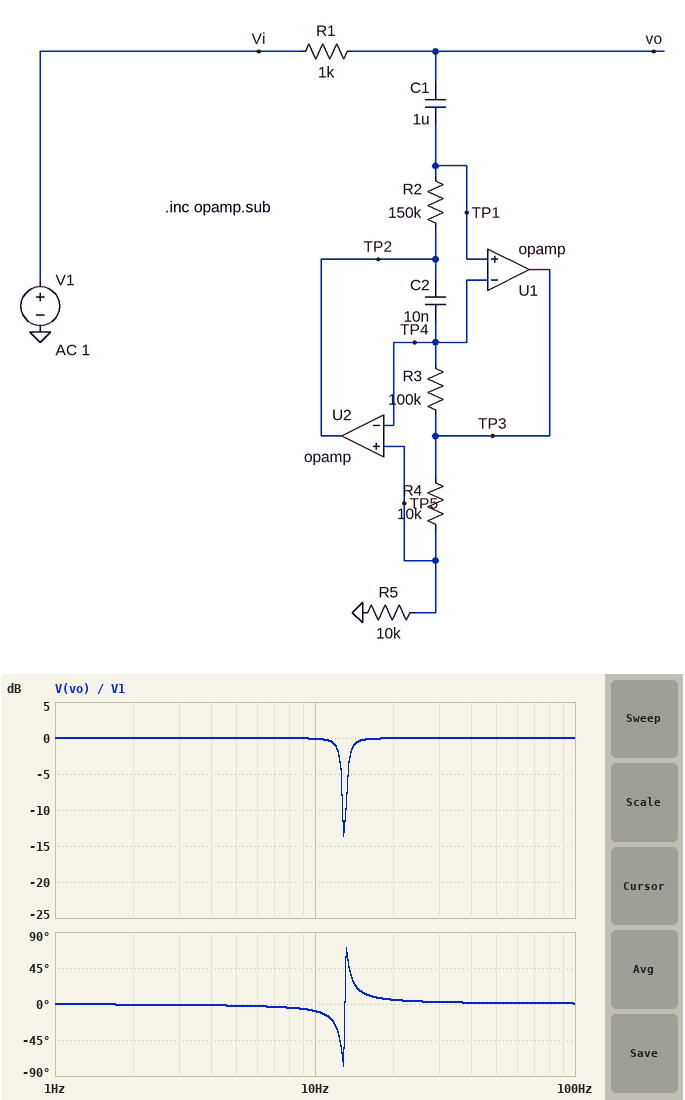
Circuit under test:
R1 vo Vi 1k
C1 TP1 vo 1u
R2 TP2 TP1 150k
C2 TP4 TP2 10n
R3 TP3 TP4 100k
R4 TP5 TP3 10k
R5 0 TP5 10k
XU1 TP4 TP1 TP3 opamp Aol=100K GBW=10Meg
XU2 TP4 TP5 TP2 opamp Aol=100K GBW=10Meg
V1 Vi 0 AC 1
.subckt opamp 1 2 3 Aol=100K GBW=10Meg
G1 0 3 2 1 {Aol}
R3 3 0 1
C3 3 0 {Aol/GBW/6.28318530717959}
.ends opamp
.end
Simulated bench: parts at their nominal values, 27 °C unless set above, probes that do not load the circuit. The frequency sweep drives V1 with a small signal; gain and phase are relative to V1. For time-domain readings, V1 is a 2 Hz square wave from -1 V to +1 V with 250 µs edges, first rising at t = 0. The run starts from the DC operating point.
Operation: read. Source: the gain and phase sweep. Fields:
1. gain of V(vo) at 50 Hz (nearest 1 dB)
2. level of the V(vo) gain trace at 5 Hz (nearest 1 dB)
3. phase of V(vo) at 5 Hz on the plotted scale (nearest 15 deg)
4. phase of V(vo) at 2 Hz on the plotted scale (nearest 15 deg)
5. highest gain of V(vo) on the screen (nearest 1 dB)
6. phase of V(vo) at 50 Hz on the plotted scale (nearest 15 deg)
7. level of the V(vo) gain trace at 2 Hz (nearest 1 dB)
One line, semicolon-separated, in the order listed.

0 dB; 0 dB; 0 deg; 0 deg; 0 dB; 0 deg; 0 dB
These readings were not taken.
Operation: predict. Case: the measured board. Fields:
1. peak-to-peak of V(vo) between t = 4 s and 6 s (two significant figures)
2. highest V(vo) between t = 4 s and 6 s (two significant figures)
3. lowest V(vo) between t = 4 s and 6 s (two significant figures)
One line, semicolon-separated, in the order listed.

2.2 V; 1.1 V; -1.1 V
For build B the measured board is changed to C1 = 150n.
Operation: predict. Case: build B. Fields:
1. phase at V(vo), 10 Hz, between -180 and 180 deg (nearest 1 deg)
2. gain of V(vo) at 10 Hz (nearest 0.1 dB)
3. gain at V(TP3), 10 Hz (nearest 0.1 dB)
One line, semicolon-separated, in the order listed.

-1 deg; 0 dB; -14.2 dB
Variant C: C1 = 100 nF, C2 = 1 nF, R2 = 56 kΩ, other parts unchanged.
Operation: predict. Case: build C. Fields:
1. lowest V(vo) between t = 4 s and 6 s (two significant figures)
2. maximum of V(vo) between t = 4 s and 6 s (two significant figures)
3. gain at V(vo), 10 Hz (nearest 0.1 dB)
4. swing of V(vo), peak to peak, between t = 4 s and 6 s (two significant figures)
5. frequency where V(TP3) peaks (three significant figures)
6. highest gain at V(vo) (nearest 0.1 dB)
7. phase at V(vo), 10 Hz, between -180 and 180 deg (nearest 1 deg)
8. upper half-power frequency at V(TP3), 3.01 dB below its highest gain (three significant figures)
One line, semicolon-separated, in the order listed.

-1.2 V; 1.2 V; 0 dB; 2.4 V; 214 Hz; 0 dB; 0 deg; 230 Hz
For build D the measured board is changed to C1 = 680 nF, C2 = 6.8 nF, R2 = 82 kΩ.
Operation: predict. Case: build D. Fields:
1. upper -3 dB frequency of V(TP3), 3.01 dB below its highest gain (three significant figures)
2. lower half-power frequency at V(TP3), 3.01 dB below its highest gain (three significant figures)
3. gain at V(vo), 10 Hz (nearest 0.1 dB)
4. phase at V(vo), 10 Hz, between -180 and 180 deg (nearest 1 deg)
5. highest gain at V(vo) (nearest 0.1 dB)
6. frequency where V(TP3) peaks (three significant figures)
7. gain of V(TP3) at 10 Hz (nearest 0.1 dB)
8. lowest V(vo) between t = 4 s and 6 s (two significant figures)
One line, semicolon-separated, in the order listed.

27.5 Hz; 24.6 Hz; 0 dB; -3 deg; 0 dB; 25.9 Hz; -9.1 dB; -1.2 V
